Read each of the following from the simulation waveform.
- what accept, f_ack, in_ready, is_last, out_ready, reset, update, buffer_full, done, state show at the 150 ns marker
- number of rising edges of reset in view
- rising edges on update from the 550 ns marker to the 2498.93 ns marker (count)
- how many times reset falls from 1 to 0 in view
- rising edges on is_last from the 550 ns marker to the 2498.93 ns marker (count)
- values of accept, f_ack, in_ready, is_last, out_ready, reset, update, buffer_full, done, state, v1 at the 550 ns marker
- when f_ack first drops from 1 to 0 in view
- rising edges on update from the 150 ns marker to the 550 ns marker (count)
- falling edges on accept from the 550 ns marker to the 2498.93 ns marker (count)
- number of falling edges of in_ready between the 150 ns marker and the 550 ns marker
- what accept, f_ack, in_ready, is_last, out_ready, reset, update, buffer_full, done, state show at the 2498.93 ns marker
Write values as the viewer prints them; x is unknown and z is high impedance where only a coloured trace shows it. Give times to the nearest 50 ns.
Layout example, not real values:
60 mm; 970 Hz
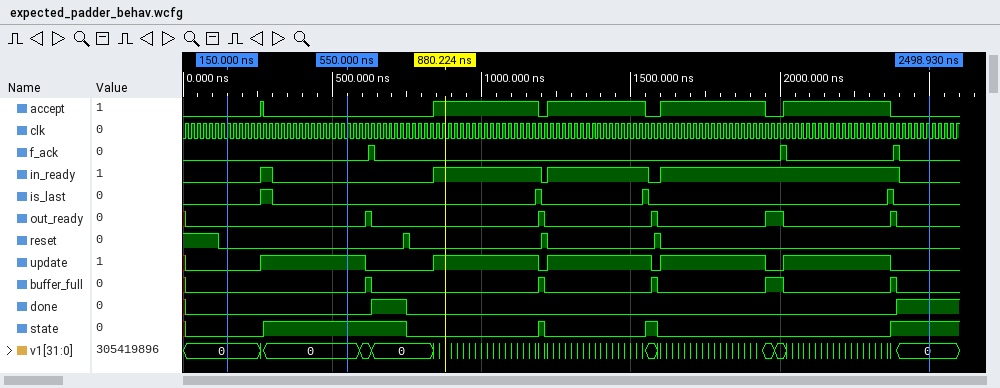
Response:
accept=0, f_ack=0, in_ready=0, is_last=0, out_ready=0, reset=0, update=0, buffer_full=0, done=0, state=0; 3; 4; 4; 3; accept=0, f_ack=0, in_ready=0, is_last=0, out_ready=0, reset=0, update=1, buffer_full=0, done=0, state=1, v1=0; 650 ns; 1; 4; 1; accept=0, f_ack=0, in_ready=0, is_last=0, out_ready=0, reset=0, update=0, buffer_full=0, done=1, state=1
